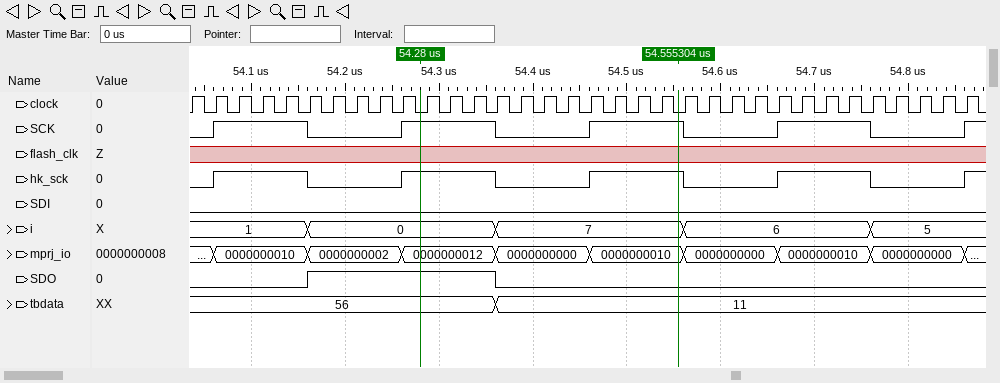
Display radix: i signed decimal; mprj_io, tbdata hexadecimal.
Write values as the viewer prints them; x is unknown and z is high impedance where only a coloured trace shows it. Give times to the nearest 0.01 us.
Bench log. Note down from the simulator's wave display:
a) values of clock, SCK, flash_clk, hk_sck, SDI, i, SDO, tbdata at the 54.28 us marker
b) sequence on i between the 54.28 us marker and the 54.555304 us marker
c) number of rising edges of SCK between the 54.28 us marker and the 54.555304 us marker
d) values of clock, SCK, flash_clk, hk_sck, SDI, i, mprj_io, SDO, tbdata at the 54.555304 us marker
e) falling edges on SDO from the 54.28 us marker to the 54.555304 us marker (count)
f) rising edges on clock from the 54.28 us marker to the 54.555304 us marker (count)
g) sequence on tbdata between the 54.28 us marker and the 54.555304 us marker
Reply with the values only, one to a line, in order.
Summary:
clock=0, SCK=1, flash_clk=x, hk_sck=1, SDI=0, i=0, SDO=1, tbdata=56
0, 7
1
clock=0, SCK=1, flash_clk=x, hk_sck=1, SDI=0, i=7, mprj_io=0000000010, SDO=0, tbdata=11
1
11
56, 11
